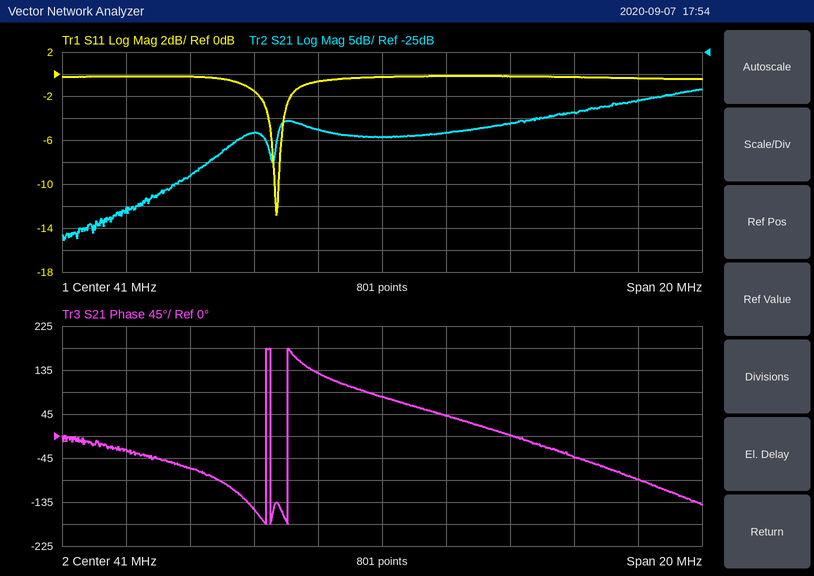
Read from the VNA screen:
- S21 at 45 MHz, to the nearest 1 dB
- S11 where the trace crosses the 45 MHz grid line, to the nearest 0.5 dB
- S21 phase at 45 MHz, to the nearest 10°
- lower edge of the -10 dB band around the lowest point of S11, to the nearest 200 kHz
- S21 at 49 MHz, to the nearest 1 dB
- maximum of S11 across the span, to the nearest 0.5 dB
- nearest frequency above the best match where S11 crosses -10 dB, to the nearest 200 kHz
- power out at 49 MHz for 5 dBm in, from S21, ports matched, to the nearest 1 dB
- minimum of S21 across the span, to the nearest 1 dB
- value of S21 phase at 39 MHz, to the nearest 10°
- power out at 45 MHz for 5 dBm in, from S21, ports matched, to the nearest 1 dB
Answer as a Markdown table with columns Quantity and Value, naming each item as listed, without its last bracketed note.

| Quantity | Value |
|---|---|
| S21 at 45 MHz, to the nearest 1 dB | -41 dB |
| S11 where the trace crosses the 45 MHz grid line, to the nearest 0.5 dB | 0.0 dB |
| S21 phase at 45 MHz, to the nearest 10° | 0° |
| lower edge of the -10 dB band around the lowest point of S11, to the nearest 200 kHz | 37.6 MHz |
| S21 at 49 MHz, to the nearest 1 dB | -36 dB |
| maximum of S11 across the span, to the nearest 0.5 dB | 0.0 dB |
| nearest frequency above the best match where S11 crosses -10 dB, to the nearest 200 kHz | 37.8 MHz |
| power out at 49 MHz for 5 dBm in, from S21, ports matched, to the nearest 1 dB | -31 dBm |
| minimum of S21 across the span, to the nearest 1 dB | -68 dB |
| value of S21 phase at 39 MHz, to the nearest 10° | 130° |
| power out at 45 MHz for 5 dBm in, from S21, ports matched, to the nearest 1 dB | -36 dBm |
